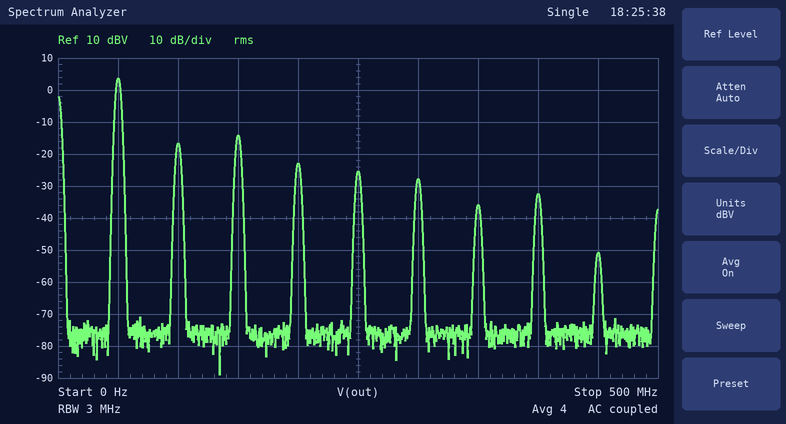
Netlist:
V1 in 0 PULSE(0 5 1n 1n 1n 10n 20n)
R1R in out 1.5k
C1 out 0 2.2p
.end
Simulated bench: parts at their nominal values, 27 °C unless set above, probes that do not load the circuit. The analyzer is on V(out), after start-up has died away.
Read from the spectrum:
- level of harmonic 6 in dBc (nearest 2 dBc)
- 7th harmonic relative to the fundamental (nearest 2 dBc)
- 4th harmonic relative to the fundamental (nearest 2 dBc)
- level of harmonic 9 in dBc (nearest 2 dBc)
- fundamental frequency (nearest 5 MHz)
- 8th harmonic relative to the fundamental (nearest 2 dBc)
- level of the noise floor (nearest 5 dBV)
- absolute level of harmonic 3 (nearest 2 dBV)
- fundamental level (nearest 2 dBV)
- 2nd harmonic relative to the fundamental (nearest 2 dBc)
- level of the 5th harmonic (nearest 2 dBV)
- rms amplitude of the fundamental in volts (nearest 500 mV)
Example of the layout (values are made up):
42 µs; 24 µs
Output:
-32 dBc; -40 dBc; -26 dBc; -54 dBc; 50 MHz; -36 dBc; -75 dBV; -14 dBV; 4 dBV; -20 dBc; -26 dBV; 1.5 V
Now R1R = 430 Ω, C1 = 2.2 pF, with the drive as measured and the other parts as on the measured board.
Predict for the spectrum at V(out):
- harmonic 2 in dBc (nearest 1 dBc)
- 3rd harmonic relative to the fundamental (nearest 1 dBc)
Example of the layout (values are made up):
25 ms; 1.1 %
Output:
-17 dBc; -13 dBc
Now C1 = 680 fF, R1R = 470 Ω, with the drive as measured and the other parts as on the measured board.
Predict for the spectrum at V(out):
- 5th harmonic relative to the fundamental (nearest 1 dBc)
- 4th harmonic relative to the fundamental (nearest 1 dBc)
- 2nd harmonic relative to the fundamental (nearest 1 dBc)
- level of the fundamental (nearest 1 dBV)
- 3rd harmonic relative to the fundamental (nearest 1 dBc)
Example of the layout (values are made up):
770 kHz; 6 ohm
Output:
-19 dBc; -18 dBc; -16 dBc; 7 dBV; -11 dBc
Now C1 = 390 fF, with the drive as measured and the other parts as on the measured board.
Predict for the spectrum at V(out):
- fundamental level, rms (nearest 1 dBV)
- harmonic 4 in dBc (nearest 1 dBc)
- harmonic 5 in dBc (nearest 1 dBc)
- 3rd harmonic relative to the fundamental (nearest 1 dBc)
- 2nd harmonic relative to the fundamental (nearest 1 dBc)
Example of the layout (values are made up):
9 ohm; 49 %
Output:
7 dBV; -19 dBc; -20 dBc; -12 dBc; -17 dBc
